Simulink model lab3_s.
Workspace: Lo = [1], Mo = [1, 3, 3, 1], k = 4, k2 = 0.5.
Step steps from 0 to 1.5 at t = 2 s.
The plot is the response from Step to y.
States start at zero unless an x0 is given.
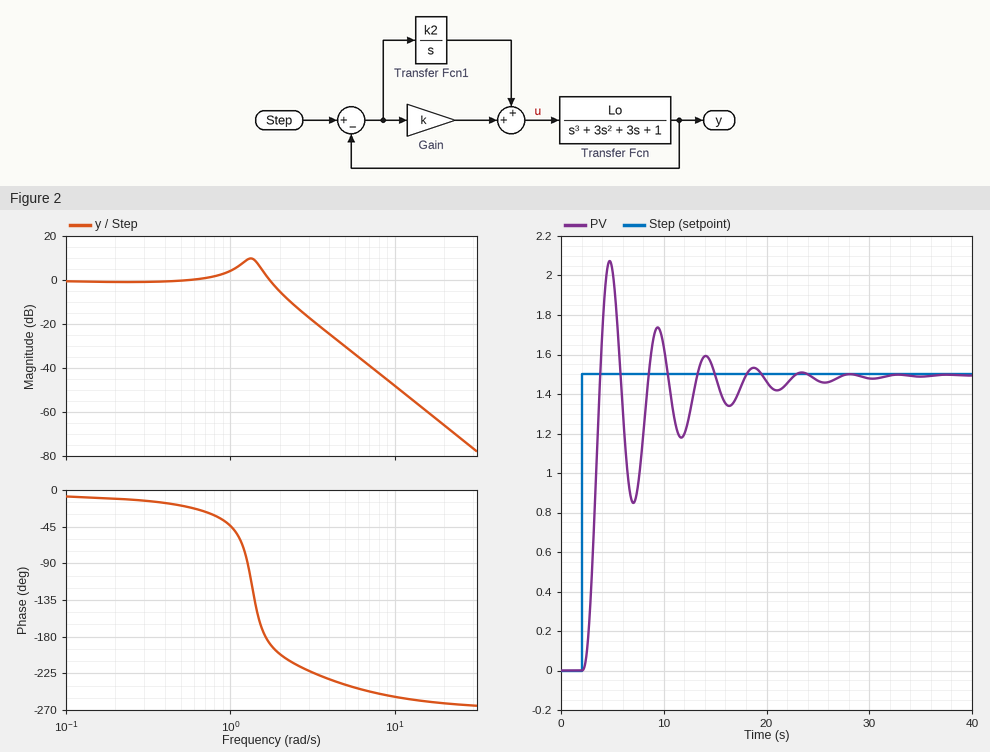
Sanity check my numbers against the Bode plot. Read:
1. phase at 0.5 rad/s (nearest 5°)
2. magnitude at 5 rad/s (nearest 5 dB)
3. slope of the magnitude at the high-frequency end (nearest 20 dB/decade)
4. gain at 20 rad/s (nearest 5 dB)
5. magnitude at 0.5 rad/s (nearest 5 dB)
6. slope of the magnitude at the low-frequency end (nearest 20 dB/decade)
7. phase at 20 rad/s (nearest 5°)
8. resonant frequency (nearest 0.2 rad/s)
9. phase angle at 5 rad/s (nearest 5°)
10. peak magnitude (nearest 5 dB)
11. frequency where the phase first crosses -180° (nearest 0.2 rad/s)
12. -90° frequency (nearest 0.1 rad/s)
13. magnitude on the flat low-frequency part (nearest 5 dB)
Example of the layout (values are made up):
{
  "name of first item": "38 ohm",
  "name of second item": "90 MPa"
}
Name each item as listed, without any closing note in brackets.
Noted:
{
  "phase at 0.5 rad/s": "-20°",
  "magnitude at 5 rad/s": "-30 dB",
  "slope of the magnitude at the high-frequency end": "-60 dB/decade",
  "gain at 20 rad/s": "-65 dB",
  "magnitude at 0.5 rad/s": "0 dB",
  "slope of the magnitude at the low-frequency end": "0 dB/decade",
  "phase at 20 rad/s": "-260°",
  "resonant frequency": "1.4 rad/s",
  "phase angle at 5 rad/s": "-240°",
  "peak magnitude": "10 dB",
  "frequency where the phase first crosses -180°": "1.6 rad/s",
  "-90° frequency": "1.3 rad/s",
  "magnitude on the flat low-frequency part": "0 dB"
}
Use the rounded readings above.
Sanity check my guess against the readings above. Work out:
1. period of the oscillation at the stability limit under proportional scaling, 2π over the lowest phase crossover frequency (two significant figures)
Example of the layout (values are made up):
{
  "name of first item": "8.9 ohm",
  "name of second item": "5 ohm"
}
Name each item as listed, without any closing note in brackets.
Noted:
{
  "period of the oscillation at the stability limit under proportional scaling, 2π over the lowest phase crossover frequency": "3.9 s"
}
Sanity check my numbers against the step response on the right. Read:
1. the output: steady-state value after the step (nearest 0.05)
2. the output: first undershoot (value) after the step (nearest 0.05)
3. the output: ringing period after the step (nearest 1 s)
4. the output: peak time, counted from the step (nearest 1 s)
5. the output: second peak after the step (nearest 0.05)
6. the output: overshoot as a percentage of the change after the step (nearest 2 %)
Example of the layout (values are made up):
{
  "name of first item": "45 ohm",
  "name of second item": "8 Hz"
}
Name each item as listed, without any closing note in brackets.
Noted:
{
  "the output: steady-state value after the step": "1.50",
  "the output: first undershoot (value) after the step": "0.85",
  "the output: ringing period after the step": "5 s",
  "the output: peak time, counted from the step": "3 s",
  "the output: second peak after the step": "1.75",
  "the output: overshoot as a percentage of the change after the step": "38 %"
}
